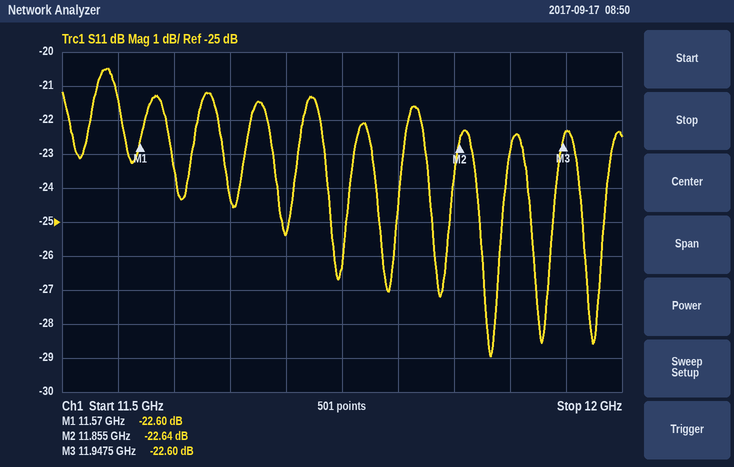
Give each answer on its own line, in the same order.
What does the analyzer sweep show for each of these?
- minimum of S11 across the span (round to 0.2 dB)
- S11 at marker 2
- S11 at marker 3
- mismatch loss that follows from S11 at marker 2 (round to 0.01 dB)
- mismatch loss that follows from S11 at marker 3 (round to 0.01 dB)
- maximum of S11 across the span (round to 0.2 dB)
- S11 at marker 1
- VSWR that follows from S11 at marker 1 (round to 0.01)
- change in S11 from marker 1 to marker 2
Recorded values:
-29.0 dB
-22.64 dB
-22.60 dB
0.02 dB
0.02 dB
-20.4 dB
-22.60 dB
1.16
-0.04 dB
